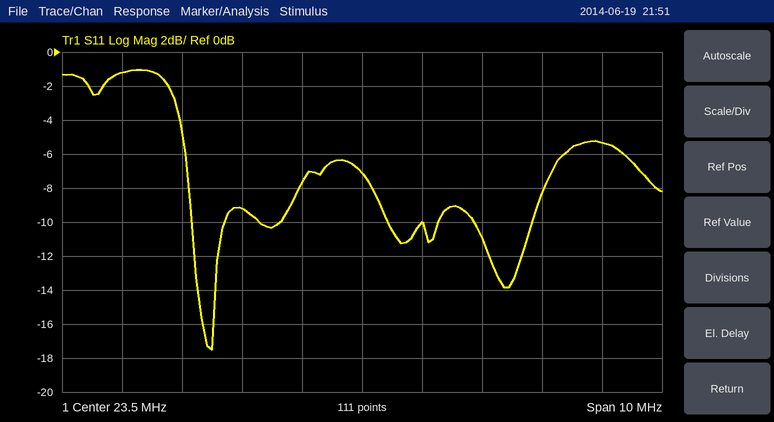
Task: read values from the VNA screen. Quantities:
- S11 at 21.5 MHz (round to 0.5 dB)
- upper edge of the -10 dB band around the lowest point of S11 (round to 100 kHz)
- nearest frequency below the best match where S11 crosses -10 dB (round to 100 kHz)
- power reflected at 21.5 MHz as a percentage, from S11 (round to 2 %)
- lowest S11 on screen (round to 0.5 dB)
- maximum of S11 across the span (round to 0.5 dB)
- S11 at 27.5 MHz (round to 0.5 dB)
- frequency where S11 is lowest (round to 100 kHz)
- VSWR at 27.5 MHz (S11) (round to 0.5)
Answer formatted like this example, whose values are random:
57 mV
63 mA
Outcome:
-9.0 dB
21.2 MHz
20.7 MHz
12 %
-17.5 dB
-1.0 dB
-5.5 dB
21.0 MHz
3.5
